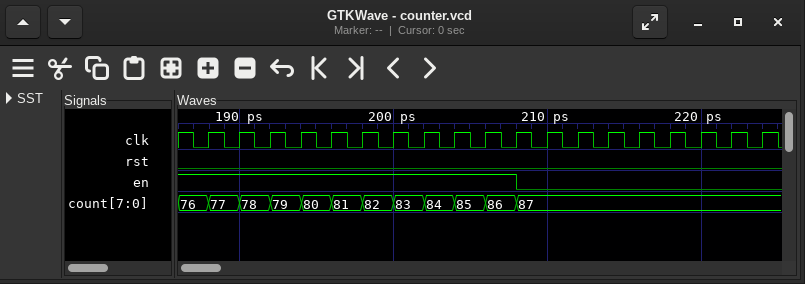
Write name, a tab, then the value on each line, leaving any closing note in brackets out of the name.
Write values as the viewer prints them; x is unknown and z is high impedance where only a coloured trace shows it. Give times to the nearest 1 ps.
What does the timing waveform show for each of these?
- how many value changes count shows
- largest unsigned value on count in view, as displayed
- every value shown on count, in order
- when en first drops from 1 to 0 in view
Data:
how many value changes count shows	11
largest unsigned value on count in view, as displayed	87
every value shown on count, in order	76, 77, 78, 79, 80, 81, 82, 83, 84, 85, 86, 87
when en first drops from 1 to 0 in view	208 ps
